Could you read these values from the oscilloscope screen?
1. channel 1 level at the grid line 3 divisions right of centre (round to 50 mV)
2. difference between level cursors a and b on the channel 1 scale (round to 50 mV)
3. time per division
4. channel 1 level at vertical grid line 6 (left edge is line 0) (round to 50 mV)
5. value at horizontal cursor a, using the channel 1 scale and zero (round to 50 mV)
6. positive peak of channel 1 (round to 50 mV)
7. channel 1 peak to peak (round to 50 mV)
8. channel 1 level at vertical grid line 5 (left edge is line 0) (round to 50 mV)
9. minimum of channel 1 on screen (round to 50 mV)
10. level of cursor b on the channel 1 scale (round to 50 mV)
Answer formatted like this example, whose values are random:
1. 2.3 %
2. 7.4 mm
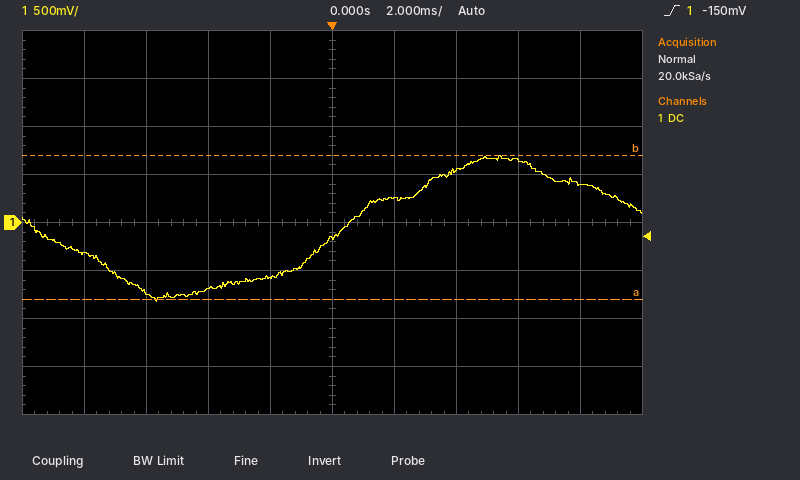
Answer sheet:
1. 650 mV
2. 1.50 V
3. 2 ms
4. 250 mV
5. -800 mV
6. 700 mV
7. 1.50 V
8. -150 mV
9. -800 mV
10. 700 mV
